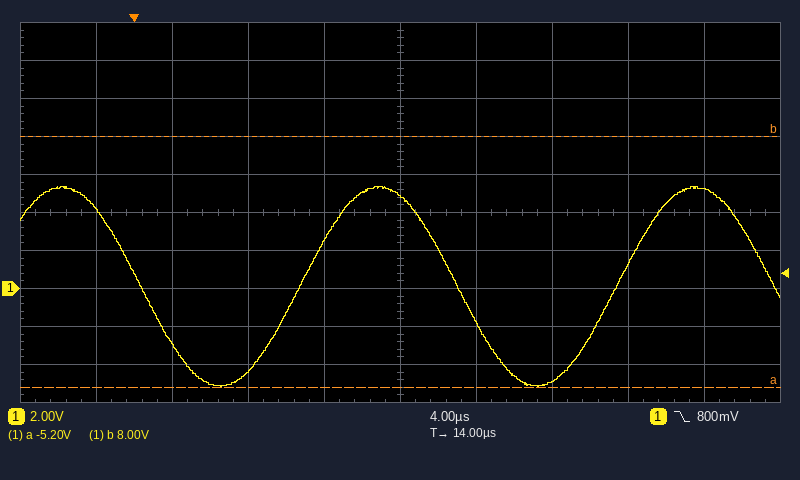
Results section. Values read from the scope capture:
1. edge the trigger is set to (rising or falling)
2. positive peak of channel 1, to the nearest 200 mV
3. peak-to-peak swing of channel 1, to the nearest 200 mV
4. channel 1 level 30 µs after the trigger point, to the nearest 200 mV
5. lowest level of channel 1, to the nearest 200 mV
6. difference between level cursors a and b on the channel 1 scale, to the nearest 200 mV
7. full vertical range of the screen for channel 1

falling
5.4 V
10.6 V
5.2 V
-5.2 V
13.2 V
20 V
